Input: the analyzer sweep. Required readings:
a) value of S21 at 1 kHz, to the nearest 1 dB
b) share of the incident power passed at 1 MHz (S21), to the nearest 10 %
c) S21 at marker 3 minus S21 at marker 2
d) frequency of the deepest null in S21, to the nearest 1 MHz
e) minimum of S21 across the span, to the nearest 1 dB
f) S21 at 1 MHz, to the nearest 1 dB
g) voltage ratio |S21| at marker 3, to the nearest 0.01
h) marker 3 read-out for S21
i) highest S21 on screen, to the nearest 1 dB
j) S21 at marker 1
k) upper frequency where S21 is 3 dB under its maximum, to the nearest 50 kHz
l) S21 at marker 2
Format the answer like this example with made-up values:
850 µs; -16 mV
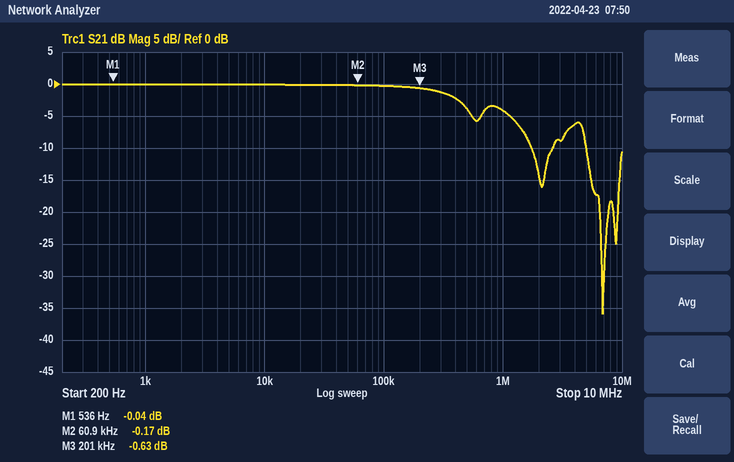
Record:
0 dB; 40 %; -0.46 dB; 7 MHz; -36 dB; -4 dB; 0.93; -0.63 dB; 0 dB; -0.04 dB; 450 kHz; -0.17 dB
